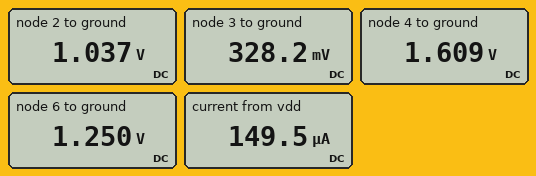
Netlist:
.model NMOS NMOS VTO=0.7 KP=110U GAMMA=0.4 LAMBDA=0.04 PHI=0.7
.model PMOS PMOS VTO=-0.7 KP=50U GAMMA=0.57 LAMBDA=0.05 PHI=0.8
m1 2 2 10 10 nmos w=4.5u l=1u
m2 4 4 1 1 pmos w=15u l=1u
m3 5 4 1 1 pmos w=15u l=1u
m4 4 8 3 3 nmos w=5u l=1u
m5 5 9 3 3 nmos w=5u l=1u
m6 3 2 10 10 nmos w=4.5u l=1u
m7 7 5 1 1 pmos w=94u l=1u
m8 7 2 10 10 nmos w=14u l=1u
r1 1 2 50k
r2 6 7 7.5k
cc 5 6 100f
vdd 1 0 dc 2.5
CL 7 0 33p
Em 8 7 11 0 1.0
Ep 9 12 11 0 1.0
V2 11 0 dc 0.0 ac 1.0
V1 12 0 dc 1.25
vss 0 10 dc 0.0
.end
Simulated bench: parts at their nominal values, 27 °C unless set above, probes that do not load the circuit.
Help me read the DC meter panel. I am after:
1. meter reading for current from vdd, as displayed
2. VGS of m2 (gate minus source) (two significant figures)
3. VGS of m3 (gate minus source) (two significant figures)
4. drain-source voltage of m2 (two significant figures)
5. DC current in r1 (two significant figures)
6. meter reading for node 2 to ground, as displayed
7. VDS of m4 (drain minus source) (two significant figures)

149.5 µA
-890 mV
-890 mV
-890 mV
29 µA
1.037 V
1.3 V
